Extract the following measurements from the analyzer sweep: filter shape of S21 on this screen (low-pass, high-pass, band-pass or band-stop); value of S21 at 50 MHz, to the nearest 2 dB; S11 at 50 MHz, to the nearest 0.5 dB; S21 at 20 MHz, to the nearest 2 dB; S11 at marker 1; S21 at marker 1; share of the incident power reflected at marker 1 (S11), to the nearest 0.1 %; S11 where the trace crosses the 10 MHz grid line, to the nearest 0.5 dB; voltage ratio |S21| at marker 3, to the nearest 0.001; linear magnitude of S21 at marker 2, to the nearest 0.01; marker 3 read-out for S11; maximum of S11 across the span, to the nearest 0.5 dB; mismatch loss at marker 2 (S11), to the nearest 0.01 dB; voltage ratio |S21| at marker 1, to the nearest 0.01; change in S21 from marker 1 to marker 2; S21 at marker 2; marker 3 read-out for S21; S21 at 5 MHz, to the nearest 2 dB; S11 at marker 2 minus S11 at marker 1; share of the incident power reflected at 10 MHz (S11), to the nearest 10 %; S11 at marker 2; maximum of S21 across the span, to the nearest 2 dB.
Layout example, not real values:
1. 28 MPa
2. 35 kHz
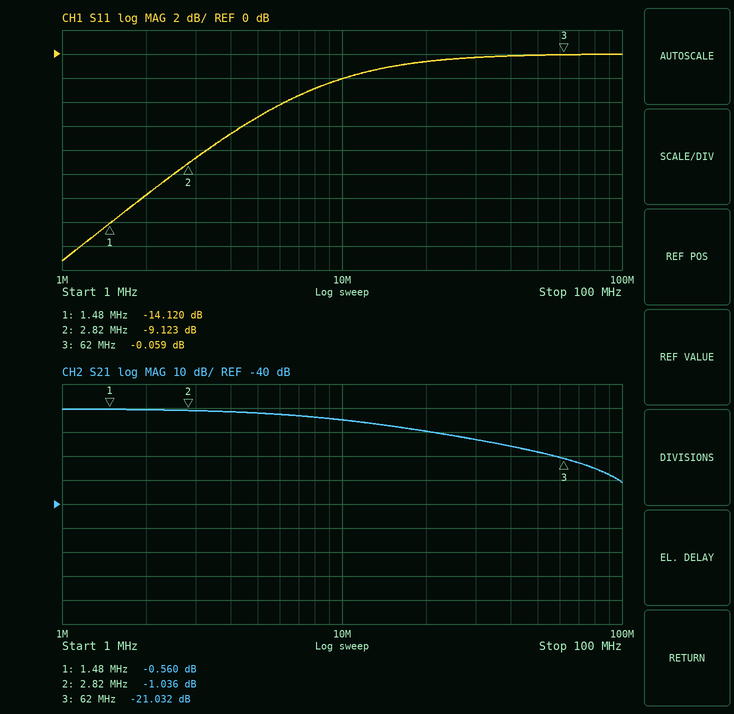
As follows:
1. low-pass
2. -18 dB
3. 0.0 dB
4. -10 dB
5. -14.120 dB
6. -0.560 dB
7. 3.9 %
8. -2.0 dB
9. 0.089
10. 0.89
11. -0.059 dB
12. 0.0 dB
13. 0.57 dB
14. 0.94
15. -0.476 dB
16. -1.036 dB
17. -21.032 dB
18. -2 dB
19. 4.997 dB
20. 60 %
21. -9.123 dB
22. 0 dB
